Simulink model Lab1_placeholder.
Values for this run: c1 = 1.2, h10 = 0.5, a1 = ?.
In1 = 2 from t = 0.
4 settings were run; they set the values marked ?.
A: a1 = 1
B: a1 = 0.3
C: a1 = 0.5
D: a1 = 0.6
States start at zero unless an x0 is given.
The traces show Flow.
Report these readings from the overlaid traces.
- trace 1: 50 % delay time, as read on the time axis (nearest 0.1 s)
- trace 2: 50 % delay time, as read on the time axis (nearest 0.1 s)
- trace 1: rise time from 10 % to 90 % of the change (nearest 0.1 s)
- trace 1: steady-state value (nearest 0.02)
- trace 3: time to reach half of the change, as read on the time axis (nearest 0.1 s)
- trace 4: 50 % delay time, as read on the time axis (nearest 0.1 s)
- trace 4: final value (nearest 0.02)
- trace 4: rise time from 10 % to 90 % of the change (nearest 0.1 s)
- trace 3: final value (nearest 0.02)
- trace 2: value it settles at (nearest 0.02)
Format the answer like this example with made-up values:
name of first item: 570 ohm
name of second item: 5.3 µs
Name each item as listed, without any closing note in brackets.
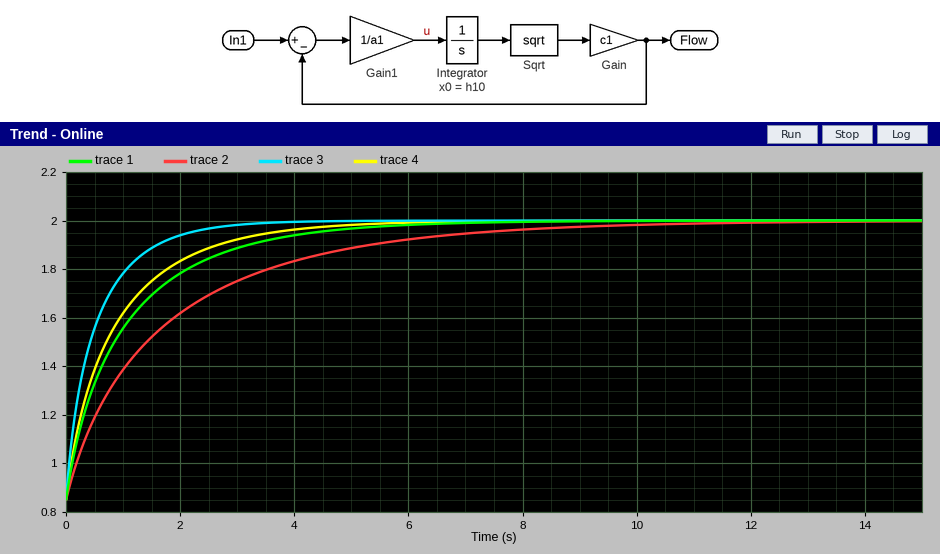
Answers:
trace 1: 50 % delay time, as read on the time axis: 0.7 s
trace 2: 50 % delay time, as read on the time axis: 1.1 s
trace 1: rise time from 10 % to 90 % of the change: 2.9 s
trace 1: steady-state value: 2.00
trace 3: time to reach half of the change, as read on the time axis: 0.3 s
trace 4: 50 % delay time, as read on the time axis: 0.6 s
trace 4: final value: 2.00
trace 4: rise time from 10 % to 90 % of the change: 2.4 s
trace 3: final value: 2.00
trace 2: value it settles at: 2.00
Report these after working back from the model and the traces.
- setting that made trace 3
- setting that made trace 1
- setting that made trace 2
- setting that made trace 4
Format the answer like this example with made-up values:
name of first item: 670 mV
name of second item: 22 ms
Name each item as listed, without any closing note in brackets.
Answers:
setting that made trace 3: B
setting that made trace 1: D
setting that made trace 2: A
setting that made trace 4: C
